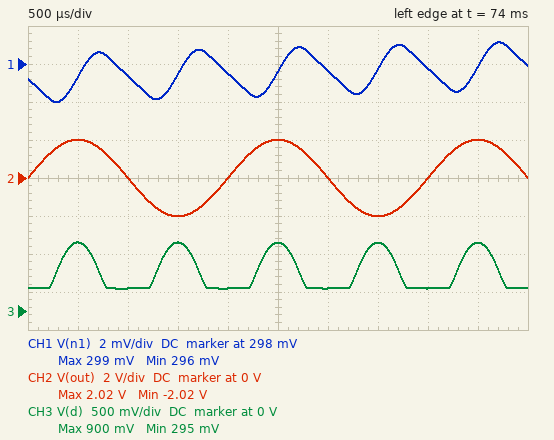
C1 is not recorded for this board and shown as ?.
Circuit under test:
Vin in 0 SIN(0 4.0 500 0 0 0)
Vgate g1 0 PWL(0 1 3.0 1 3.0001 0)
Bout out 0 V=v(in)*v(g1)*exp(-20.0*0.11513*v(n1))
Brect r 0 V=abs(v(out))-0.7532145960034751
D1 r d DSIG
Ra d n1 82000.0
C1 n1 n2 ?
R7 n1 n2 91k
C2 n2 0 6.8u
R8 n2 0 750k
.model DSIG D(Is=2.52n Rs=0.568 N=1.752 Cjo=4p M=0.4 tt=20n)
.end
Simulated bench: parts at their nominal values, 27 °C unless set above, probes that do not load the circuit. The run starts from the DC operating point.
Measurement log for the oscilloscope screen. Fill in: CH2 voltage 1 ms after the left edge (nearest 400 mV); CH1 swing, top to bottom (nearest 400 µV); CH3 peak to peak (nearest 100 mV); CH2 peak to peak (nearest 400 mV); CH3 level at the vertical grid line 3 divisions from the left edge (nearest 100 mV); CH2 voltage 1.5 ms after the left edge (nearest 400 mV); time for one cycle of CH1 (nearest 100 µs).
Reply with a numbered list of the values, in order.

1. 0 V
2. 3.2 mV
3. 600 mV
4. 4.0 V
5. 900 mV
6. -2.0 V
7. 1.0 ms
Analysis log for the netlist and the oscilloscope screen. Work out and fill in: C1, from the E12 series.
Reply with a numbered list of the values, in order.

1. 560 nF
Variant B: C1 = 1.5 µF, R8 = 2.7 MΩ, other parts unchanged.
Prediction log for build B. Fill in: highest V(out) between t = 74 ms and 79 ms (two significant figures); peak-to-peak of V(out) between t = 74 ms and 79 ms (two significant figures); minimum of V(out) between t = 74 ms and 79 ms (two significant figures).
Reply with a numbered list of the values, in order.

1. 2.1 V
2. 4.1 V
3. -2.1 V
